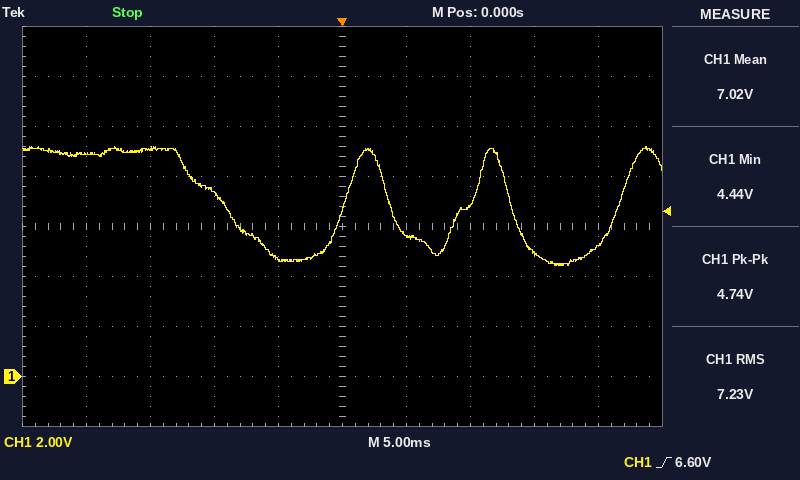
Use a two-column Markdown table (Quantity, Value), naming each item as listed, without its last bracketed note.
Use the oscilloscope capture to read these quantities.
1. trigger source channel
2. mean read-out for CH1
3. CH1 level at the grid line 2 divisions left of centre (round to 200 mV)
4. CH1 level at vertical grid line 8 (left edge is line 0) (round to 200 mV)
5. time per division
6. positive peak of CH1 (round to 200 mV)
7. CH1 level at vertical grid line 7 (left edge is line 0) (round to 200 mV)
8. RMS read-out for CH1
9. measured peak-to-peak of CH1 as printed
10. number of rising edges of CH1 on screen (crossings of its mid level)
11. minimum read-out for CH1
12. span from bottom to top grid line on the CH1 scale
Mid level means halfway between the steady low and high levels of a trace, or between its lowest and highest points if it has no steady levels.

| Quantity | Value |
|---|---|
| trigger source channel | CH1 |
| mean read-out for CH1 | 7.02 V |
| CH1 level at the grid line 2 divisions left of centre | 7.4 V |
| CH1 level at vertical grid line 8 (left edge is line 0) | 5.0 V |
| time per division | 5 ms |
| positive peak of CH1 | 9.2 V |
| CH1 level at vertical grid line 7 (left edge is line 0) | 6.8 V |
| RMS read-out for CH1 | 7.23 V |
| measured peak-to-peak of CH1 as printed | 4.74 V |
| number of rising edges of CH1 on screen | 3 |
| minimum read-out for CH1 | 4.44 V |
| span from bottom to top grid line on the CH1 scale | 16 V |
